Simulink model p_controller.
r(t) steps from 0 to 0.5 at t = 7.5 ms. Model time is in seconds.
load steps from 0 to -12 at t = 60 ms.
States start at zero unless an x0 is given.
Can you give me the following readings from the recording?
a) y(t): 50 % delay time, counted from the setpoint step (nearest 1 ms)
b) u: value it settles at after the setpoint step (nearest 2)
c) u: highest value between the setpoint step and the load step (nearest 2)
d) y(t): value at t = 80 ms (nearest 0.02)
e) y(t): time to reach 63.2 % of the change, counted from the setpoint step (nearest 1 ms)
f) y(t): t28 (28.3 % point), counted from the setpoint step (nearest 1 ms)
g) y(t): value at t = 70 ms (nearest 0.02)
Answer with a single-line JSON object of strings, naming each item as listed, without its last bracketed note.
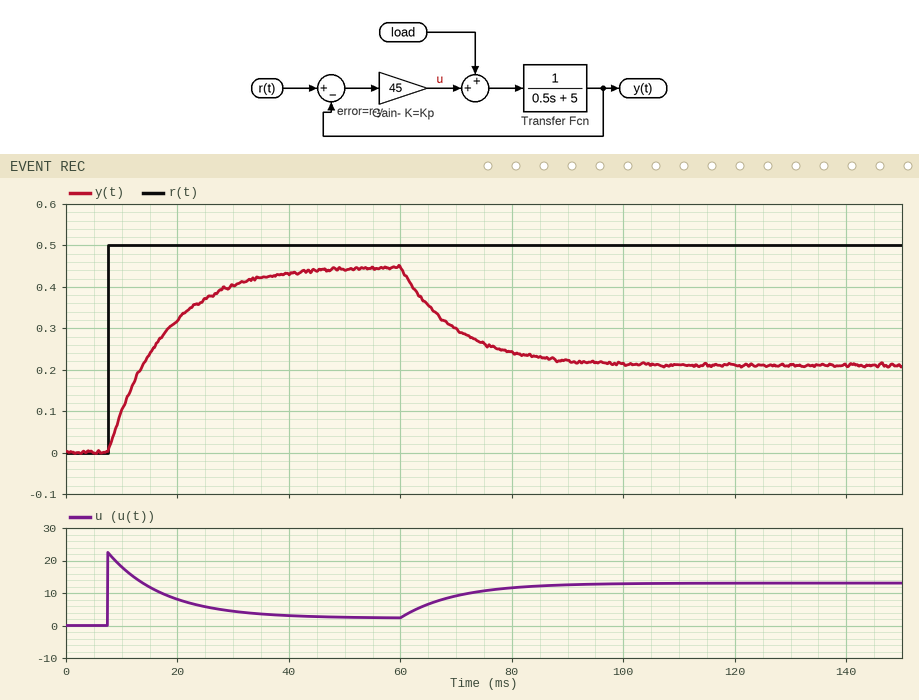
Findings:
{"y(t): 50 % delay time, counted from the setpoint step": "7 ms", "u: value it settles at after the setpoint step": "2", "u: highest value between the setpoint step and the load step": "22", "y(t): value at t = 80 ms": "0.24", "y(t): time to reach 63.2 % of the change, counted from the setpoint step": "10 ms", "y(t): t28 (28.3 % point), counted from the setpoint step": "3 ms", "y(t): value at t = 70 ms": "0.30"}
